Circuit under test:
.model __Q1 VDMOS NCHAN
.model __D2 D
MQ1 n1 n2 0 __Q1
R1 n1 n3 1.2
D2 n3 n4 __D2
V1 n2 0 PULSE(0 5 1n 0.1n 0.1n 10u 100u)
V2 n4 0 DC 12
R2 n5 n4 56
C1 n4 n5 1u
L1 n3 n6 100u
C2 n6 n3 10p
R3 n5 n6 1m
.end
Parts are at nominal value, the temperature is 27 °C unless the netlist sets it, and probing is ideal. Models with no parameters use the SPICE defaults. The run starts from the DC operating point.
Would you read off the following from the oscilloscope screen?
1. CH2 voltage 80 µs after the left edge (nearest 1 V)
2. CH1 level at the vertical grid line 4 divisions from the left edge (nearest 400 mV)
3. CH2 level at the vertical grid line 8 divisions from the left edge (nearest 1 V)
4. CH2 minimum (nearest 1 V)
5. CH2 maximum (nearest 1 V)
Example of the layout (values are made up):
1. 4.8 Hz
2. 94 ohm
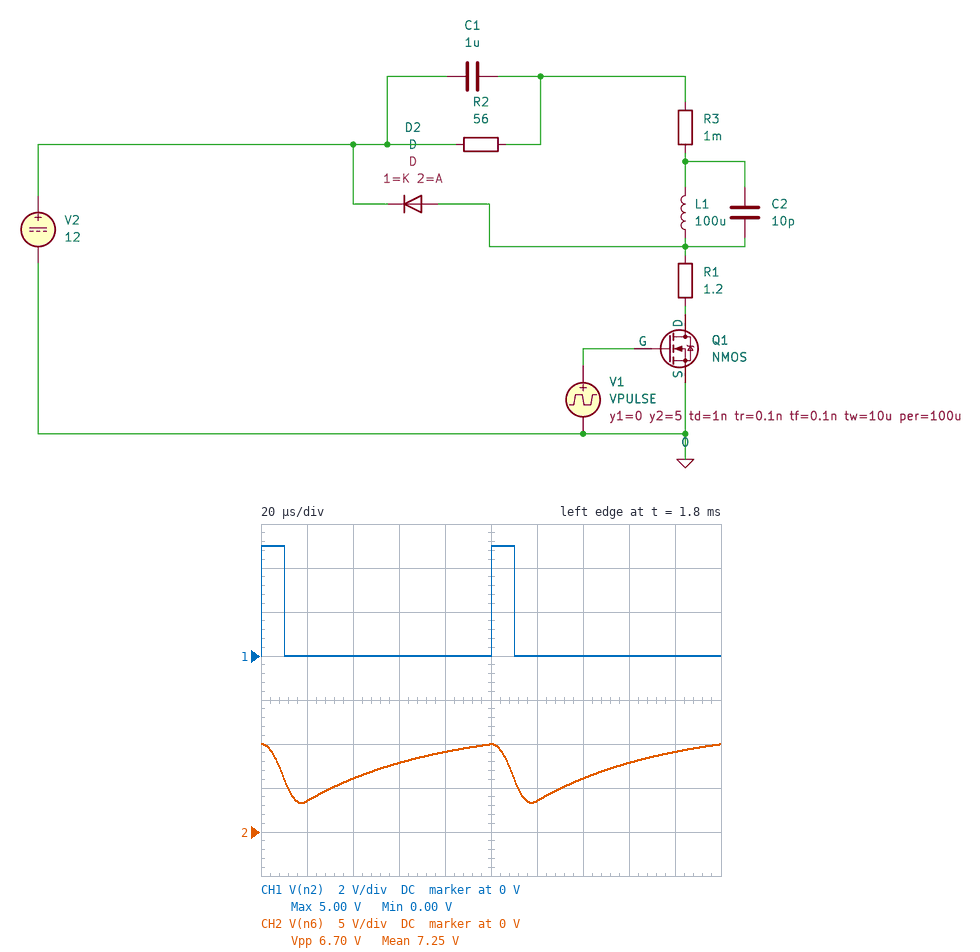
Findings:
1. 9 V
2. 0 V
3. 8 V
4. 3 V
5. 10 V
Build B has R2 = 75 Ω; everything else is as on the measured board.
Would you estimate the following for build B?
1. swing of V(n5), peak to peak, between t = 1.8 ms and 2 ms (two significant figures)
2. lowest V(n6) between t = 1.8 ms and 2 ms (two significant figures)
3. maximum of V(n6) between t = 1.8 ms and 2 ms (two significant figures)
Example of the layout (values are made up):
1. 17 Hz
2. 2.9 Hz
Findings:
1. 5.9 V
2. 3.2 V
3. 9.1 V
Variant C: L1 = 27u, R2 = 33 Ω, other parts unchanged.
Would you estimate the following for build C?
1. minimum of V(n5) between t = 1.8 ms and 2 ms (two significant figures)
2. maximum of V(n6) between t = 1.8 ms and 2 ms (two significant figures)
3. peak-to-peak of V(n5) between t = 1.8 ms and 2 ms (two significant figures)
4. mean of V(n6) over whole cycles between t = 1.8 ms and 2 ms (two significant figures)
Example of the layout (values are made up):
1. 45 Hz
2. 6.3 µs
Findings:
1. -2.3 V
2. 11 V
3. 13 V
4. 6.8 V
